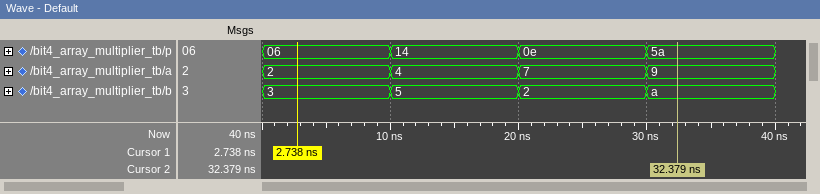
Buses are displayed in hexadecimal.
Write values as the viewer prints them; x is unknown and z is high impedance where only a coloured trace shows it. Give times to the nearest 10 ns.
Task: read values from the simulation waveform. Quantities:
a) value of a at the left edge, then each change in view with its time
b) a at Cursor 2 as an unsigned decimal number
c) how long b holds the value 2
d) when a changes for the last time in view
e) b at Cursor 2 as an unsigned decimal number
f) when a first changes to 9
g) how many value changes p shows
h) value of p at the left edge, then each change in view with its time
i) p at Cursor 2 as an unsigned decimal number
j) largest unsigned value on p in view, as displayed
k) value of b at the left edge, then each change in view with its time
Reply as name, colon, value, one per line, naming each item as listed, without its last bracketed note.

value of a at the left edge, then each change in view with its time: 2, 4 at 10 ns, 7 at 20 ns, 9 at 30 ns
a at Cursor 2 as an unsigned decimal number: 9
how long b holds the value 2: 10 ns
when a changes for the last time in view: 30 ns
b at Cursor 2 as an unsigned decimal number: 10
when a first changes to 9: 30 ns
how many value changes p shows: 3
value of p at the left edge, then each change in view with its time: 06, 14 at 10 ns, 0e at 20 ns, 5a at 30 ns
p at Cursor 2 as an unsigned decimal number: 90
largest unsigned value on p in view, as displayed: 5a
value of b at the left edge, then each change in view with its time: 3, 5 at 10 ns, 2 at 20 ns, a at 30 ns
